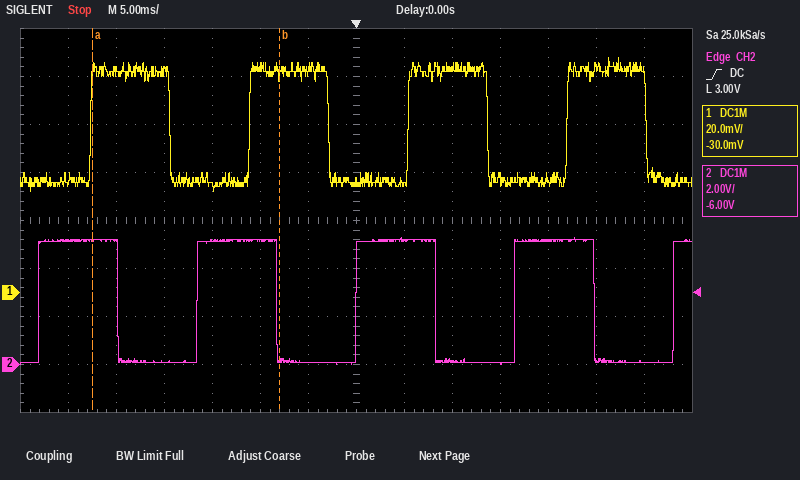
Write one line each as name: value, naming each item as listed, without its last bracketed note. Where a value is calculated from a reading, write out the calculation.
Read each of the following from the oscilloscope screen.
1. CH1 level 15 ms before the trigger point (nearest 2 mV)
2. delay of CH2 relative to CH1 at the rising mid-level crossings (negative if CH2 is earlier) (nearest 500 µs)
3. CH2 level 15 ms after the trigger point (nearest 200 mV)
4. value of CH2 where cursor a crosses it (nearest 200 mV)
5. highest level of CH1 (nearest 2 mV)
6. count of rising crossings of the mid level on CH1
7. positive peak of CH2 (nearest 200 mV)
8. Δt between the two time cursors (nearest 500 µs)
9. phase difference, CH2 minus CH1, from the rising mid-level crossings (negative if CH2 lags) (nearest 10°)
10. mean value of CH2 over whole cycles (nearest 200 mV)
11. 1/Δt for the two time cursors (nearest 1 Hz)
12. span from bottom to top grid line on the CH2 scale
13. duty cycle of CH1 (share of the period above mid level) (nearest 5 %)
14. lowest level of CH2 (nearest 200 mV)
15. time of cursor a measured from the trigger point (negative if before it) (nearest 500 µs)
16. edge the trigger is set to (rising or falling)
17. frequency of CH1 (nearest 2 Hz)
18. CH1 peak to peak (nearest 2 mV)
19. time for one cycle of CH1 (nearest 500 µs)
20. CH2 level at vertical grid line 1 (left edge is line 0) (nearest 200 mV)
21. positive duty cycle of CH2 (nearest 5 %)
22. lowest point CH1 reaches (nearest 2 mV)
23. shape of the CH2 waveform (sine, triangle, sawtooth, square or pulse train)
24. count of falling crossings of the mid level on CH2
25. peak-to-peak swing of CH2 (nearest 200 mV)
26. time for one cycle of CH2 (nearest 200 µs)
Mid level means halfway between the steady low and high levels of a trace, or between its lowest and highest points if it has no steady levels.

CH1 level 15 ms before the trigger point: 44 mV
delay of CH2 relative to CH1 at the rising mid-level crossings (negative if CH2 is earlier): -5.5 ms
CH2 level 15 ms after the trigger point: 0.0 V
value of CH2 where cursor a crosses it: 5.2 V
highest level of CH1: 98 mV
count of rising crossings of the mid level on CH1: 4
positive peak of CH2: 5.2 V
Δt between the two time cursors: 19.5 ms
phase difference, CH2 minus CH1, from the rising mid-level crossings (negative if CH2 lags): −360° × (-5.5 ms) / 16.5 ms ≈ +120°
mean value of CH2 over whole cycles: 0.0 V + 0.5 × (5.2 V − (0.0 V)) ≈ 2.6 V
1/Δt for the two time cursors: 1 / 19.5 ms ≈ 51 Hz
span from bottom to top grid line on the CH2 scale: 16 V
duty cycle of CH1 (share of the period above mid level): 50 %
lowest level of CH2: 0.0 V
time of cursor a measured from the trigger point (negative if before it): -27.5 ms
edge the trigger is set to: rising
frequency of CH1: 1 / 16.5 ms ≈ 60.6 Hz, so 60 Hz to the nearest 2 Hz
CH1 peak to peak: 98 mV − (42 mV) = 56 mV
time for one cycle of CH1: 16.5 ms
CH2 level at vertical grid line 1 (left edge is line 0): 5.2 V
positive duty cycle of CH2: 50 %
lowest point CH1 reaches: 42 mV
shape of the CH2 waveform: square
count of falling crossings of the mid level on CH2: 4
peak-to-peak swing of CH2: 5.2 V − (0.0 V) = 5.2 V
time for one cycle of CH2: 16.6 ms
